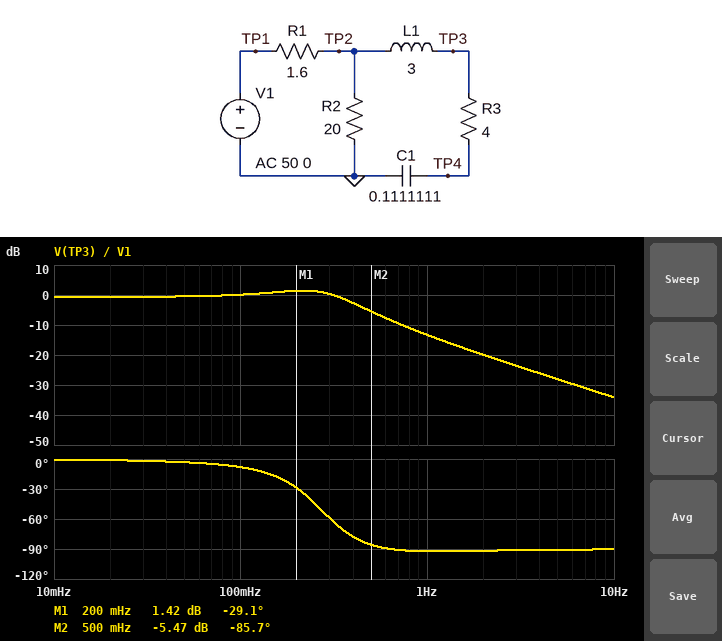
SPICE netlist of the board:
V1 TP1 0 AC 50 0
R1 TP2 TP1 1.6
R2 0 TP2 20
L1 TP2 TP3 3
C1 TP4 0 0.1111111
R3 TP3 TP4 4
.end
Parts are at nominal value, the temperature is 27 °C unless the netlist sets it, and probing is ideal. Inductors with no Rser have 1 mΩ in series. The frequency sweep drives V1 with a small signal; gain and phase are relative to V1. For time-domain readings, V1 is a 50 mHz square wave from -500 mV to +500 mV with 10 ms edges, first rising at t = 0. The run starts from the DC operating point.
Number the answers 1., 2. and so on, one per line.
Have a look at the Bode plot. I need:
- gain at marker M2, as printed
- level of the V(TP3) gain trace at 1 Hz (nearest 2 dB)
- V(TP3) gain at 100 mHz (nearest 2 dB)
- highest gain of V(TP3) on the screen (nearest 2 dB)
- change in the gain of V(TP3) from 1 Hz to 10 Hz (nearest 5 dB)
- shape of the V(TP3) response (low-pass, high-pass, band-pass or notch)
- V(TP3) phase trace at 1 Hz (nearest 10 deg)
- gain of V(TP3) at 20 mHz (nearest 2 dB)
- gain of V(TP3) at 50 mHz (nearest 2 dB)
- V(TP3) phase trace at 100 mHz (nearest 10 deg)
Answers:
1. -5.47 dB
2. -14 dB
3. 0 dB
4. 2 dB
5. -20 dB
6. low-pass
7. -90 deg
8. 0 dB
9. 0 dB
10. -10 deg
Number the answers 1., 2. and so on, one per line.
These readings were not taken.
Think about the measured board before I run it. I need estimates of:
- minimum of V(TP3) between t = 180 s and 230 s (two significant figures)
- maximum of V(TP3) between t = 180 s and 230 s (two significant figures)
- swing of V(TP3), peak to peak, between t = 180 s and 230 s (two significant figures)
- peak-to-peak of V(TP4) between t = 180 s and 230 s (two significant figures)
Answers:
1. -660 mV
2. 660 mV
3. 1.3 V
4. 1.2 V
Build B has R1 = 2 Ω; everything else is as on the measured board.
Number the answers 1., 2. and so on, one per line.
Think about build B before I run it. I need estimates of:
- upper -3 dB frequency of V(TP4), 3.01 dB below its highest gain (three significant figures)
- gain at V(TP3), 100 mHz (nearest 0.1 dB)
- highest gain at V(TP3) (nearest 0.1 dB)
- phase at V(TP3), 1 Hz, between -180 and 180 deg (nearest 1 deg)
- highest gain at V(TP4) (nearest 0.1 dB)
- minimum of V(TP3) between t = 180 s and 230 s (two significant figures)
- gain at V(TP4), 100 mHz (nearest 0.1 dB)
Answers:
1. 314 mHz
2. -0.1 dB
3. 0.9 dB
4. -91 deg
5. -0.2 dB
6. -620 mV
7. -0.5 dB
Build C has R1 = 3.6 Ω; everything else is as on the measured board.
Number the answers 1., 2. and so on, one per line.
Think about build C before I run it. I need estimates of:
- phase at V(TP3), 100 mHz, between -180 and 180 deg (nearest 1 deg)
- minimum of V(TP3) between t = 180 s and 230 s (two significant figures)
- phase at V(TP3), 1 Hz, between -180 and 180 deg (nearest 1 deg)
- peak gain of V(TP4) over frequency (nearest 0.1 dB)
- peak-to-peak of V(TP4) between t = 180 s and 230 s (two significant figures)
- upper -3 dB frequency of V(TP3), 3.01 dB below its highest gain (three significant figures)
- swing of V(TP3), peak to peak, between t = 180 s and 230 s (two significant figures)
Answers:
1. -14 deg
2. -500 mV
3. -88 deg
4. -1.4 dB
5. 940 mV
6. 356 mHz
7. 1.0 V
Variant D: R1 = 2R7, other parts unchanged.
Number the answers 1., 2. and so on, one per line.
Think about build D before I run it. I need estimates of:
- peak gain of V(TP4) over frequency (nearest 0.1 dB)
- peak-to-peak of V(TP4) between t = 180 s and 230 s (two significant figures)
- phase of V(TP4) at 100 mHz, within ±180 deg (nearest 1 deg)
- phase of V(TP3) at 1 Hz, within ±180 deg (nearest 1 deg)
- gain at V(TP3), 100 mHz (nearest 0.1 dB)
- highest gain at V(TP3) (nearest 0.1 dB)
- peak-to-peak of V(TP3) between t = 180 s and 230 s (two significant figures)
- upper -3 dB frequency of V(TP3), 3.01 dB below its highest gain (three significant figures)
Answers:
1. -0.8 dB
2. 1.0 V
3. -27 deg
4. -90 deg
5. -0.6 dB
6. 0 dB
7. 1.1 V
8. 362 mHz
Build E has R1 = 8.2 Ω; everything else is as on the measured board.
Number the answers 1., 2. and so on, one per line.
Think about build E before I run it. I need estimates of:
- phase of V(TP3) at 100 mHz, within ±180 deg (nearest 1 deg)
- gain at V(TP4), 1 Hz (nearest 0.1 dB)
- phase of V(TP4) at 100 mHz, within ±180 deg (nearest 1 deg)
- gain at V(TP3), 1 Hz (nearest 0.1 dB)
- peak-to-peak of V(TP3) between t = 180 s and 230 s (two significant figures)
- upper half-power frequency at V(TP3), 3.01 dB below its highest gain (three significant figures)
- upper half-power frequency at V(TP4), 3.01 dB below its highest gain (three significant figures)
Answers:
1. -23 deg
2. -25.9 dB
3. -38 deg
4. -16.4 dB
5. 710 mV
6. 251 mHz
7. 192 mHz
